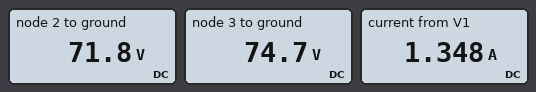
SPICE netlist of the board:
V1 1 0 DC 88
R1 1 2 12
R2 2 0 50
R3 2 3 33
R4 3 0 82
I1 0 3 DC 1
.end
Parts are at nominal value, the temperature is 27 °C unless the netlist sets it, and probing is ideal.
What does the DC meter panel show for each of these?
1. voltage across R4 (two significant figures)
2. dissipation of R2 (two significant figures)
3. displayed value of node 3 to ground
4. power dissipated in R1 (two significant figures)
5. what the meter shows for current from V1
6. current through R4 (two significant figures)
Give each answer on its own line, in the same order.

75 V
100 W
74.7 V
22 W
1.348 A
910 mA
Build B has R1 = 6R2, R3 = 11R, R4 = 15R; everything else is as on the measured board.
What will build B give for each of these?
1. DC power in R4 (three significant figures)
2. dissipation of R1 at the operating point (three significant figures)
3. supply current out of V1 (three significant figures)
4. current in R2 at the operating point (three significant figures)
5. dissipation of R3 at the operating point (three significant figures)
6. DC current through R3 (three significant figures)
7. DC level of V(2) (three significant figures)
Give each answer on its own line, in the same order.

136 W
69.7 W
3.35 A
1.34 A
44.4 W
2.01 A
67.2 V
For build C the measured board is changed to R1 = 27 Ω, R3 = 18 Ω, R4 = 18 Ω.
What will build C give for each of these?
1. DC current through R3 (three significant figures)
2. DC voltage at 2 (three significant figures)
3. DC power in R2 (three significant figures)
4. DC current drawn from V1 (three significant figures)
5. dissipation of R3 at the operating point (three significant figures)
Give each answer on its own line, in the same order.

731 mA
44.3 V
39.3 W
1.62 A
9.62 W
